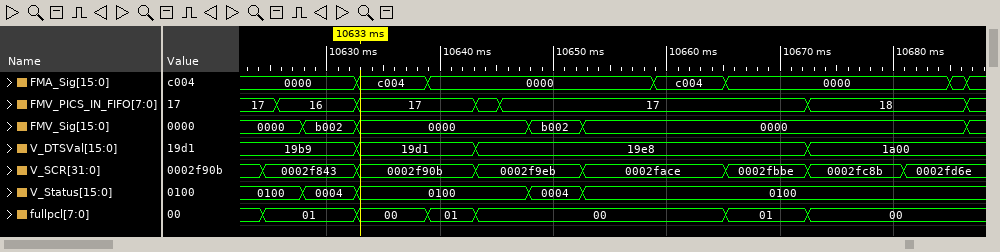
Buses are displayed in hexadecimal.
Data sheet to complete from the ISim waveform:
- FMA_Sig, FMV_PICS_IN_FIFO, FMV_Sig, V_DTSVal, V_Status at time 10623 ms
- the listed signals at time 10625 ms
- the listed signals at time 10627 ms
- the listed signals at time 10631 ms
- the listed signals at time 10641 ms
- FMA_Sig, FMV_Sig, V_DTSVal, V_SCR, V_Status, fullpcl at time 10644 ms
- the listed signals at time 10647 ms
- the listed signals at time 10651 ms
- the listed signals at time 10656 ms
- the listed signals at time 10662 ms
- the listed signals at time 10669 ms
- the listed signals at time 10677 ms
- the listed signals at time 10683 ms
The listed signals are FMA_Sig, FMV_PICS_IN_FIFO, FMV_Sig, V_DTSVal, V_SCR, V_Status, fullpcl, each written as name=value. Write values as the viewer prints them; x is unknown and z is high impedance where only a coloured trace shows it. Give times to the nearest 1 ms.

FMA_Sig=0000, FMV_PICS_IN_FIFO=17, FMV_Sig=0000, V_DTSVal=19b9, V_Status=0100
FMA_Sig=0000, FMV_PICS_IN_FIFO=17, FMV_Sig=0000, V_DTSVal=19b9, V_SCR=0002f843, V_Status=0100, fullpcl=01
FMA_Sig=0000, FMV_PICS_IN_FIFO=16, FMV_Sig=0000, V_DTSVal=19b9, V_SCR=0002f843, V_Status=0100, fullpcl=01
FMA_Sig=0000, FMV_PICS_IN_FIFO=16, FMV_Sig=b002, V_DTSVal=19b9, V_SCR=0002f843, V_Status=0004, fullpcl=01
FMA_Sig=0000, FMV_PICS_IN_FIFO=17, FMV_Sig=0000, V_DTSVal=19d1, V_SCR=0002f90b, V_Status=0100, fullpcl=01
FMA_Sig=0000, FMV_Sig=0000, V_DTSVal=19e8, V_SCR=0002f9eb, V_Status=0100, fullpcl=00
FMA_Sig=0000, FMV_PICS_IN_FIFO=17, FMV_Sig=0000, V_DTSVal=19e8, V_SCR=0002f9eb, V_Status=0100, fullpcl=00
FMA_Sig=0000, FMV_PICS_IN_FIFO=17, FMV_Sig=b002, V_DTSVal=19e8, V_SCR=0002f9eb, V_Status=0004, fullpcl=00
FMA_Sig=0000, FMV_PICS_IN_FIFO=17, FMV_Sig=0000, V_DTSVal=19e8, V_SCR=0002face, V_Status=0100, fullpcl=00
FMA_Sig=c004, FMV_PICS_IN_FIFO=17, FMV_Sig=0000, V_DTSVal=19e8, V_SCR=0002face, V_Status=0100, fullpcl=00
FMA_Sig=0000, FMV_PICS_IN_FIFO=17, FMV_Sig=0000, V_DTSVal=19e8, V_SCR=0002fbbe, V_Status=0100, fullpcl=01
FMA_Sig=0000, FMV_PICS_IN_FIFO=18, FMV_Sig=0000, V_DTSVal=1a00, V_SCR=0002fc8b, V_Status=0100, fullpcl=00
FMA_Sig=0000, FMV_PICS_IN_FIFO=18, FMV_Sig=0000, V_DTSVal=1a00, V_SCR=0002fd6e, V_Status=0100, fullpcl=00
